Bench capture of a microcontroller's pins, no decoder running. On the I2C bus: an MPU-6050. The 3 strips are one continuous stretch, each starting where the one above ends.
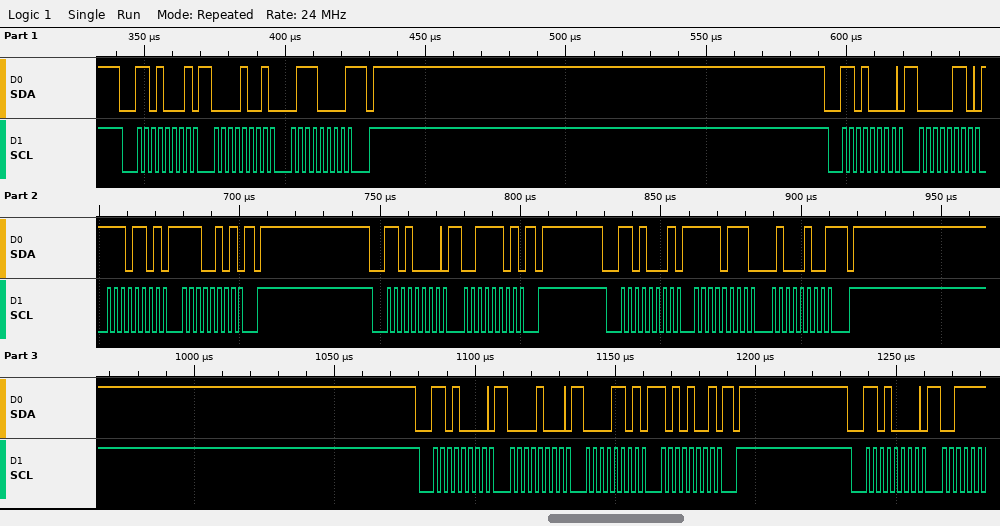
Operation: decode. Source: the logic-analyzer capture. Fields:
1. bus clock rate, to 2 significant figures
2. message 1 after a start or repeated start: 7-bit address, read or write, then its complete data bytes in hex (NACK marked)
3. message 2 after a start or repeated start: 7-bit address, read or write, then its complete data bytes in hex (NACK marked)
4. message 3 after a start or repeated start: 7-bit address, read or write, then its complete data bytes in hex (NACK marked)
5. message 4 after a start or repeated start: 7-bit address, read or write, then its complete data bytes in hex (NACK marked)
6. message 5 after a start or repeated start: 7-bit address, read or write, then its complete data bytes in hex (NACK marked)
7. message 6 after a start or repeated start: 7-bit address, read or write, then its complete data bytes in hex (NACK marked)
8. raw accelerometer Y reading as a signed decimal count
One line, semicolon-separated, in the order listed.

400 kHz; 0x68 read: 09 70 NACK; 0x68 write: 06 ED E5; 0x68 write: 3D; 0x68 read: F7 44 NACK; 0x68 write: 08 0D A9; 0x68 write; -2236
